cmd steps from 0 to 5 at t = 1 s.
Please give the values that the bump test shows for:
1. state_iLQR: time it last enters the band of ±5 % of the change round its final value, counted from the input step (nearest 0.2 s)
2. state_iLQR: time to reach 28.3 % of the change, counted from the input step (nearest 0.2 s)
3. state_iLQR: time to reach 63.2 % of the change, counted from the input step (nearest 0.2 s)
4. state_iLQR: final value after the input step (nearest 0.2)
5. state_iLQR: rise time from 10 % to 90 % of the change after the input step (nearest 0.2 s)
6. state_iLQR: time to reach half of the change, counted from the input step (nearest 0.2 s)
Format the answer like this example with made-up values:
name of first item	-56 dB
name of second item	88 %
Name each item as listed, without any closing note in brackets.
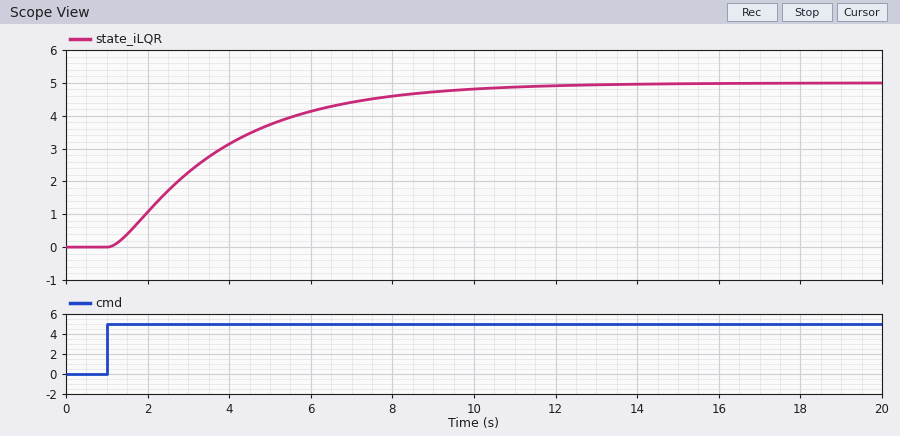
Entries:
state_iLQR: time it last enters the band of ±5 % of the change round its final value, counted from the input step	8.2 s
state_iLQR: time to reach 28.3 % of the change, counted from the input step	1.2 s
state_iLQR: time to reach 63.2 % of the change, counted from the input step	3.0 s
state_iLQR: final value after the input step	5.0
state_iLQR: rise time from 10 % to 90 % of the change after the input step	5.8 s
state_iLQR: time to reach half of the change, counted from the input step	2.2 s
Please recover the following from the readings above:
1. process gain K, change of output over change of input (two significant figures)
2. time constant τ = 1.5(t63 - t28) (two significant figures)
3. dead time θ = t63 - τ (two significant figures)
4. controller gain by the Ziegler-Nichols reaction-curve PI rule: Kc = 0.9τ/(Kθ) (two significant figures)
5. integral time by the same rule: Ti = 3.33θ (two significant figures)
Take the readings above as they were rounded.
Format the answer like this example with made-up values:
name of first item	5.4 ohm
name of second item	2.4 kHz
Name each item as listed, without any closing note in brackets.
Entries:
process gain K, change of output over change of input	1.0
time constant τ = 1.5(t63 - t28)	2.7 s
dead time θ = t63 - τ	0.30 s
controller gain by the Ziegler-Nichols reaction-curve PI rule: Kc = 0.9τ/(Kθ)	8.1
integral time by the same rule: Ti = 3.33θ	1.00 s
